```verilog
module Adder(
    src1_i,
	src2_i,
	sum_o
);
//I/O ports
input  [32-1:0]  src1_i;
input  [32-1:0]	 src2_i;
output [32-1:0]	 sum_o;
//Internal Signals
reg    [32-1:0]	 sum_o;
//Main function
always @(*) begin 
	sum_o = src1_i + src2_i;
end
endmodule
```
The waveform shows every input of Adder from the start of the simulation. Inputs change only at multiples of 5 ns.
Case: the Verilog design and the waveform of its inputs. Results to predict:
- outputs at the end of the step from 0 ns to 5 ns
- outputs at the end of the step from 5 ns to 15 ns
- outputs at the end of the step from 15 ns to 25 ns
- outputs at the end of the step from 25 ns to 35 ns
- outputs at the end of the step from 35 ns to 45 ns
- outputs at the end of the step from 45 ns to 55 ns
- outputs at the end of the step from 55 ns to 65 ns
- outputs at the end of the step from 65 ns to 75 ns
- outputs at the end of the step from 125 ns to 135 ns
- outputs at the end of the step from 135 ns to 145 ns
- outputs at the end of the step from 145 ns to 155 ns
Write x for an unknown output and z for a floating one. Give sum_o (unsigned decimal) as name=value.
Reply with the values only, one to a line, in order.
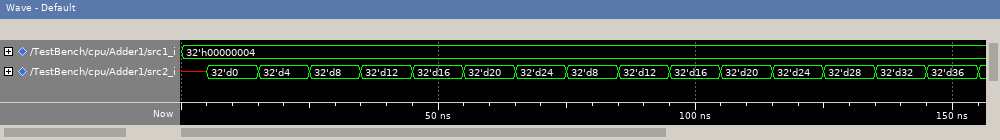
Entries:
sum_o=x
sum_o=4
sum_o=8
sum_o=12
sum_o=16
sum_o=20
sum_o=24
sum_o=28
sum_o=32
sum_o=36
sum_o=40
